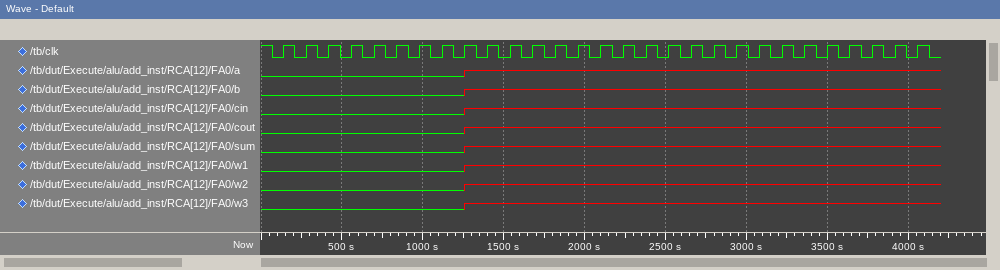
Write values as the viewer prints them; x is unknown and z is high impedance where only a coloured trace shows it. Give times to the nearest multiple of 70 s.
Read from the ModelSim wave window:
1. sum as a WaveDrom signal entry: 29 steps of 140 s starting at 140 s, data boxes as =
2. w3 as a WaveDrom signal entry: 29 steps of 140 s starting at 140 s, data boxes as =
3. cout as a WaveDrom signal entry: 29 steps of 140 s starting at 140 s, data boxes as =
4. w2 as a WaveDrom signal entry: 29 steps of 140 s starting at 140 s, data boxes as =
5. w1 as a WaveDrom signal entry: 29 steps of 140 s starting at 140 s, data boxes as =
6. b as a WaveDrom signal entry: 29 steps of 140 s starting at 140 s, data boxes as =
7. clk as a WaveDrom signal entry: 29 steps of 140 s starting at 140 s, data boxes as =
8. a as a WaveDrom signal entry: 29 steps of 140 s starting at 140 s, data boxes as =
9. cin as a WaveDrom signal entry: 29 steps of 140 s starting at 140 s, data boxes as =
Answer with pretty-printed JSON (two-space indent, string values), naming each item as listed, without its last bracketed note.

{
  "sum as a WaveDrom signal entry: 29 steps of 140 s starting at 140 s, data boxes as =": "{name: 'sum', wave: '0.......x....................'}",
  "w3 as a WaveDrom signal entry: 29 steps of 140 s starting at 140 s, data boxes as =": "{name: 'w3', wave: '0.......x....................'}",
  "cout as a WaveDrom signal entry: 29 steps of 140 s starting at 140 s, data boxes as =": "{name: 'cout', wave: '0.......x....................'}",
  "w2 as a WaveDrom signal entry: 29 steps of 140 s starting at 140 s, data boxes as =": "{name: 'w2', wave: '0.......x....................'}",
  "w1 as a WaveDrom signal entry: 29 steps of 140 s starting at 140 s, data boxes as =": "{name: 'w1', wave: '0.......x....................'}",
  "b as a WaveDrom signal entry: 29 steps of 140 s starting at 140 s, data boxes as =": "{name: 'b', wave: '0.......x....................'}",
  "clk as a WaveDrom signal entry: 29 steps of 140 s starting at 140 s, data boxes as =": "{name: 'clk', wave: 'p............................'}",
  "a as a WaveDrom signal entry: 29 steps of 140 s starting at 140 s, data boxes as =": "{name: 'a', wave: '0.......x....................'}",
  "cin as a WaveDrom signal entry: 29 steps of 140 s starting at 140 s, data boxes as =": "{name: 'cin', wave: '0.......x....................'}"
}
